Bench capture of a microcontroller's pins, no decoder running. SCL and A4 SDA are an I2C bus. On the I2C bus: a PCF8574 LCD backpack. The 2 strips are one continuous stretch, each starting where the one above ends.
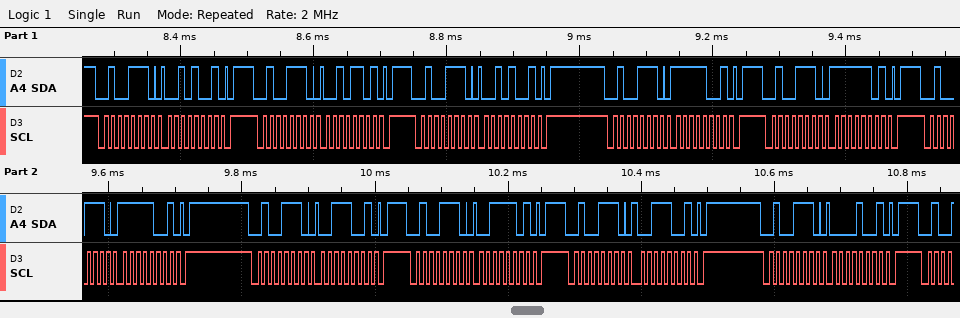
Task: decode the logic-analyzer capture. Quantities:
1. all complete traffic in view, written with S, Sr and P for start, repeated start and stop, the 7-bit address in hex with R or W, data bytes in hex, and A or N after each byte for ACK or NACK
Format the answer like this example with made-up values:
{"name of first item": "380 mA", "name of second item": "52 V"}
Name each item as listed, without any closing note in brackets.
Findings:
{"all complete traffic in view, written with S, Sr and P for start, repeated start and stop, the 7-bit address in hex with R or W, data bytes in hex, and A or N after each byte for ACK or NACK": "S 27W A 29 A P S 27W A 2D A P S 27W A 29 A P S 27W A F9 A P S 27W A FD A P S 27W A F9 A P S 27W A 39 A P S 27W A 3D A P S 27W A 39 A P S 27W A 09 A P"}
